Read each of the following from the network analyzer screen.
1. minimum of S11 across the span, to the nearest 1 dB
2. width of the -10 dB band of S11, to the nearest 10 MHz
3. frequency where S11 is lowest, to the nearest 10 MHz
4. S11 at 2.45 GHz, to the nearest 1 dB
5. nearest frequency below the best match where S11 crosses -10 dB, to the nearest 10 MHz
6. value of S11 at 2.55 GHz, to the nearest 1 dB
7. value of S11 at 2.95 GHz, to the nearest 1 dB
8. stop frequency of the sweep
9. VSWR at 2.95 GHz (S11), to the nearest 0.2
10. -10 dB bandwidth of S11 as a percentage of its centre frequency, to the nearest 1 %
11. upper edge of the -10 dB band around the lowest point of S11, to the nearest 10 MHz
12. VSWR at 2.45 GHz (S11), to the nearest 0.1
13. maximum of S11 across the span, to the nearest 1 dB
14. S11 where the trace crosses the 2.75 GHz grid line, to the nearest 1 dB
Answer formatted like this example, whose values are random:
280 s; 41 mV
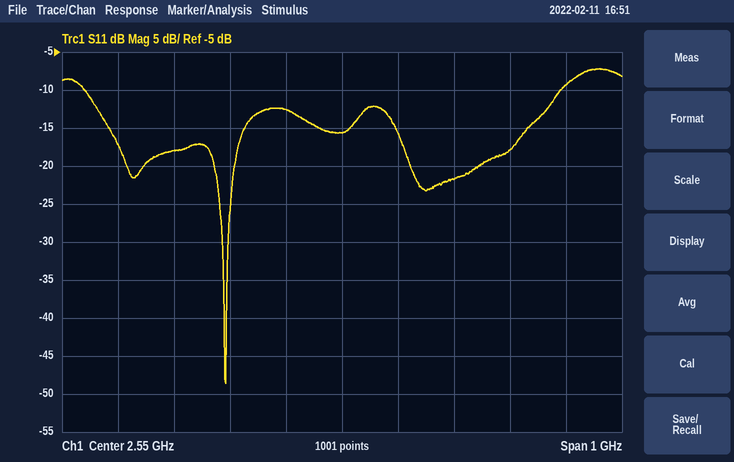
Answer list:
-49 dB; 850 MHz; 2.34 GHz; -13 dB; 2.09 GHz; -16 dB; -9 dB; 3.05 GHz; 2.0; 34 %; 2.94 GHz; 1.6; -7 dB; -22 dB
